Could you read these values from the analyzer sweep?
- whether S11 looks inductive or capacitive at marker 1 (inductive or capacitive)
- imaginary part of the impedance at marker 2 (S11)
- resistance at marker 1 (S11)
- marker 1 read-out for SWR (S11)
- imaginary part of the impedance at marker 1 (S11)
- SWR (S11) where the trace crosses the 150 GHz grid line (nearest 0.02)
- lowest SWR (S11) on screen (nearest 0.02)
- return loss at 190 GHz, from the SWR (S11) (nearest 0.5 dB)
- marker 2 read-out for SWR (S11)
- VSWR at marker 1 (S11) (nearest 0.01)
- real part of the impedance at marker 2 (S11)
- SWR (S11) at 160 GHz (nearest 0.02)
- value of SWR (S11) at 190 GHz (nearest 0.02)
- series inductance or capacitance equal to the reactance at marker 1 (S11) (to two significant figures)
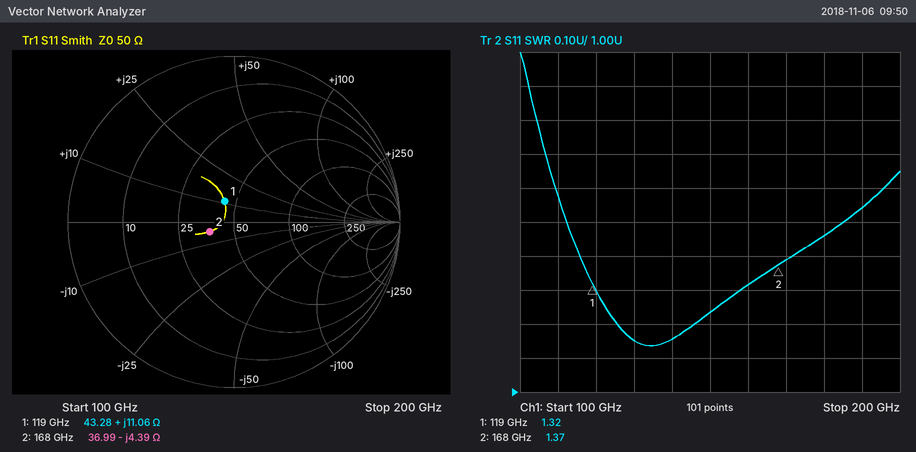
inductive
-4.39 Ω
43.28 Ω
1.32
+11.06 Ω
1.24
1.14
13.5 dB
1.37
1.32
36.99 Ω
1.32
1.54
15 pH
